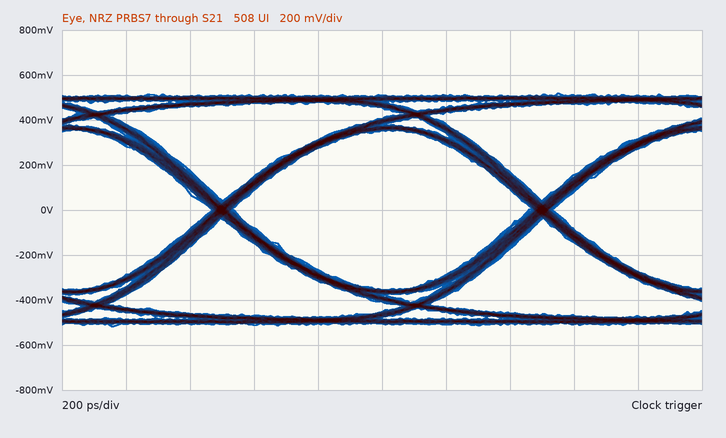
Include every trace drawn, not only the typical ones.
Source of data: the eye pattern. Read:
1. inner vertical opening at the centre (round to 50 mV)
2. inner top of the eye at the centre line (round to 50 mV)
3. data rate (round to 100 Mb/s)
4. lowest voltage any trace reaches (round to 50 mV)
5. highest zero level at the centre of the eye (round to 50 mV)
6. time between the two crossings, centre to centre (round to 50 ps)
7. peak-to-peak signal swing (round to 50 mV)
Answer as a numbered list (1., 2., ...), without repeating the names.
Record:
1. 700 mV
2. 350 mV
3. 1.0 Gb/s
4. -500 mV
5. -350 mV
6. 1.00 ns
7. 1.05 V
